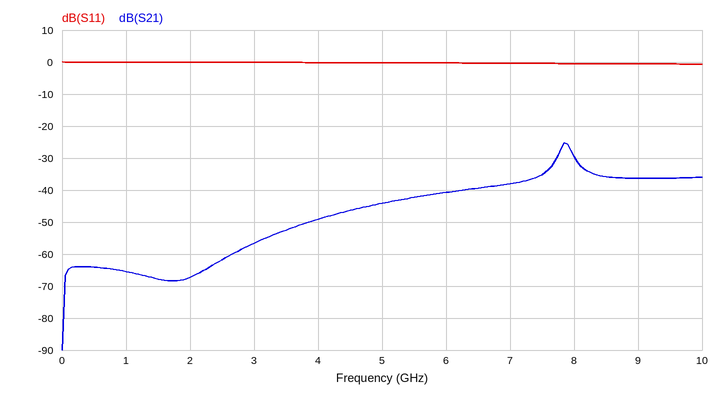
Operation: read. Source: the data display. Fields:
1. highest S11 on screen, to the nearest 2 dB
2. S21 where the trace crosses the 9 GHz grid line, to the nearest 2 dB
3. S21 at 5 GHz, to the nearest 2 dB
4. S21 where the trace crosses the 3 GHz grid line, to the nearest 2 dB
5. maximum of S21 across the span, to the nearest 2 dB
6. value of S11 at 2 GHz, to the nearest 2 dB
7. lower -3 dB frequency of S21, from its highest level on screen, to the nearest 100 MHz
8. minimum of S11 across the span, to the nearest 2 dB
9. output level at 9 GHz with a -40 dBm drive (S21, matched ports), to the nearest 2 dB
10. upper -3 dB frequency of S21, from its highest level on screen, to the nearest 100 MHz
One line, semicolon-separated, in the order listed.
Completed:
0 dB; -36 dB; -44 dB; -56 dB; -26 dB; 0 dB; 7.8 GHz; 0 dB; -76 dBm; 8.0 GHz
